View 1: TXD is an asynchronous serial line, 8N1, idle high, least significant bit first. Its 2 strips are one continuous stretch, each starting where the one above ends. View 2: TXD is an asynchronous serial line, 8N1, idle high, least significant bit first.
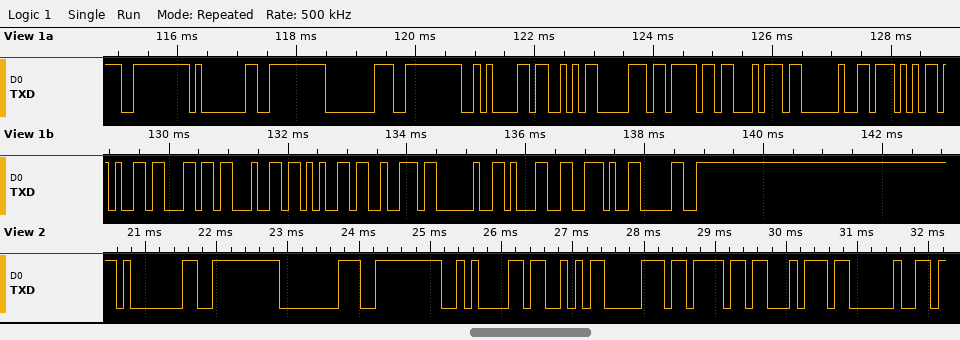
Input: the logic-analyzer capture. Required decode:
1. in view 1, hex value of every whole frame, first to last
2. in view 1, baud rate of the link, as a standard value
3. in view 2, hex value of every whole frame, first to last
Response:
FE 01 FE 80 FE 0A 53 70 6F 74 20 57 65 6C 64 65 72 20 31 2E 30
9600 baud
01 FE 80 FE 0A 53 70 6F 74 20
